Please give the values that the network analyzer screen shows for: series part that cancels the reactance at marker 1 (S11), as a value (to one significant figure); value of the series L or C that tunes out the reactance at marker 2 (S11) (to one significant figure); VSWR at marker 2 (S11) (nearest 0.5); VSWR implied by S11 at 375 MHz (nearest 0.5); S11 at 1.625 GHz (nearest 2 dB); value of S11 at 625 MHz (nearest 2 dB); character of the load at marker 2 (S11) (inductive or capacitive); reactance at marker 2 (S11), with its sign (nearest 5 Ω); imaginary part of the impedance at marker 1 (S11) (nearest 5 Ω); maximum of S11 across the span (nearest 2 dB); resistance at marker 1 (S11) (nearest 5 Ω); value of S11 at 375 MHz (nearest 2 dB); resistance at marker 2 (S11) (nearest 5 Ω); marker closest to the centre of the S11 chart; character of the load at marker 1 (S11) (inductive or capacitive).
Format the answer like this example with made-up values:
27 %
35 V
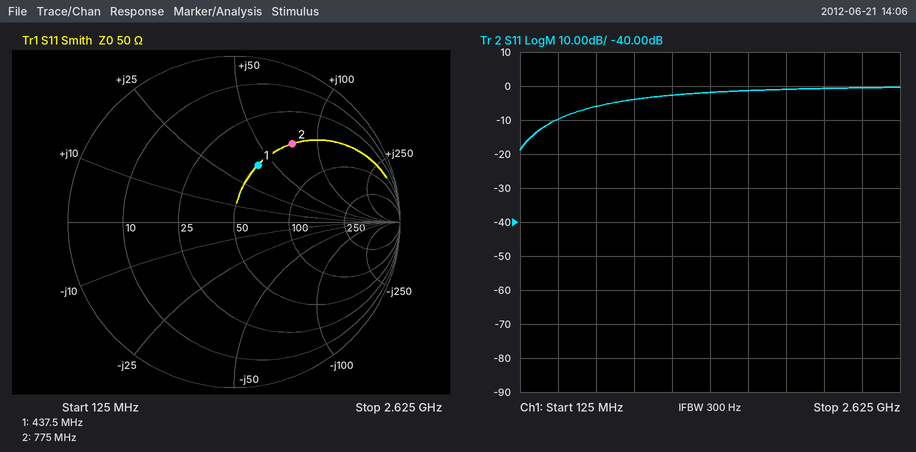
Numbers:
9 pF
3 pF
4.0
2.0
-2 dB
-6 dB
inductive
+75 Ω
+40 Ω
0 dB
50 Ω
-10 dB
50 Ω
marker 1
inductive
